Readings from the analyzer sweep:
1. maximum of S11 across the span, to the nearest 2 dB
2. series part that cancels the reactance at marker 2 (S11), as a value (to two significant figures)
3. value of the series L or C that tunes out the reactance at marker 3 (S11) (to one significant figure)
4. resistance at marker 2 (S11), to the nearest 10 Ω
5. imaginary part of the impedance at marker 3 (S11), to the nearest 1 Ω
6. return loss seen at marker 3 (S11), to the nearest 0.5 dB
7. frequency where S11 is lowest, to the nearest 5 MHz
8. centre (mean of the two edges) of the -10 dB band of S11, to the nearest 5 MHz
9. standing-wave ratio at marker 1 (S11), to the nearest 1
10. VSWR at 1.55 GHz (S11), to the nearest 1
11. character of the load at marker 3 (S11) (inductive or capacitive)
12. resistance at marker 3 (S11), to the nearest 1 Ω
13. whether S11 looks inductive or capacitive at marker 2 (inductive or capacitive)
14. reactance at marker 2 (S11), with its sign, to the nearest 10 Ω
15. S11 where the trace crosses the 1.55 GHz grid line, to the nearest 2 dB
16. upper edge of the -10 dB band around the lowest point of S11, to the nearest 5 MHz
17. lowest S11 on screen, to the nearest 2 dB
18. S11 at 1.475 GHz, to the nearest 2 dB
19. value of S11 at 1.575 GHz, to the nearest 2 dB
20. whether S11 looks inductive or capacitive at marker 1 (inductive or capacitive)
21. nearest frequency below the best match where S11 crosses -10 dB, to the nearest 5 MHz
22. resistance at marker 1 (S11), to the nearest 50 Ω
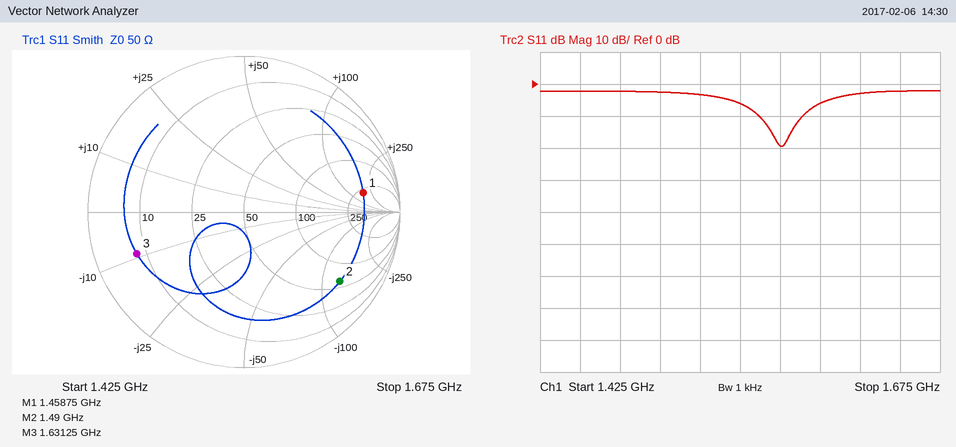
-2 dB
14 nH
900 pH
60 Ω
-9 Ω
2.5 dB
1.575 GHz
1.575 GHz
8
3
capacitive
8 Ω
capacitive
-130 Ω
-6 dB
1.590 GHz
-20 dB
-2 dB
-20 dB
inductive
1.560 GHz
300 Ω
